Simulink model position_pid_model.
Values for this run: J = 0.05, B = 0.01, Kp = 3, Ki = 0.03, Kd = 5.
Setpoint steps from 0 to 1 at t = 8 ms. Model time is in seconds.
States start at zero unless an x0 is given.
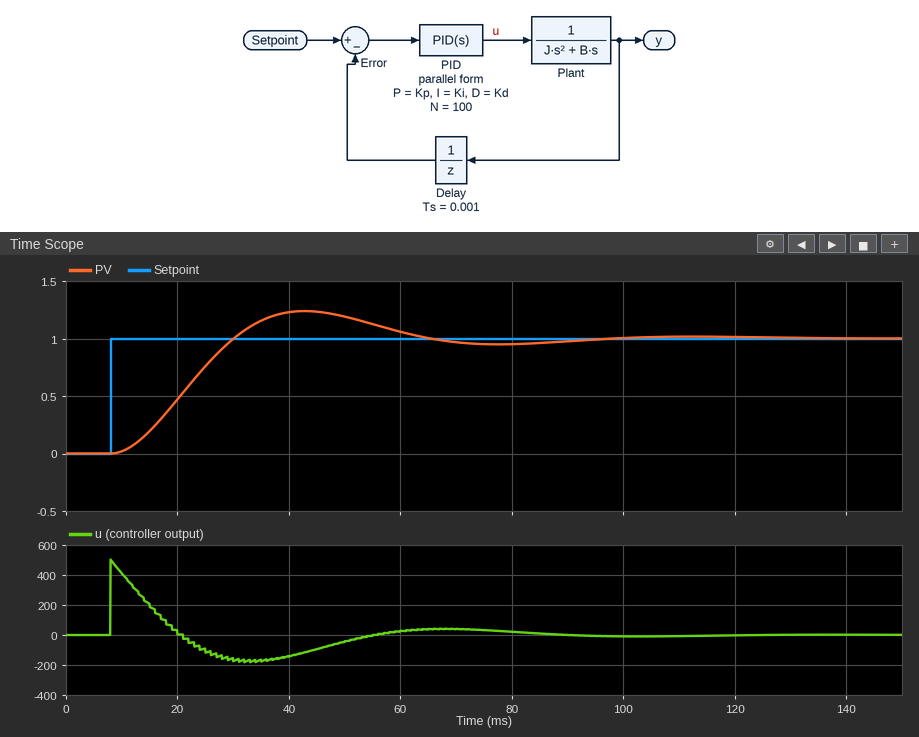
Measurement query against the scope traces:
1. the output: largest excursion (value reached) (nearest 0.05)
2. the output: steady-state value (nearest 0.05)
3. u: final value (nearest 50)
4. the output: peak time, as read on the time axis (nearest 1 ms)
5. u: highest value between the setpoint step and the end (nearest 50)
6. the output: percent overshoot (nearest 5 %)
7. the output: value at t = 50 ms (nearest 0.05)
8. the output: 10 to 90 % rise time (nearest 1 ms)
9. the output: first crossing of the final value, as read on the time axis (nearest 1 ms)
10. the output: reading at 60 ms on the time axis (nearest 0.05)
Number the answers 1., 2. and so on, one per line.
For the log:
1. 1.25
2. 1.00
3. 0
4. 43 ms
5. 500
6. 25 %
7. 1.20
8. 15 ms
9. 30 ms
10. 1.05
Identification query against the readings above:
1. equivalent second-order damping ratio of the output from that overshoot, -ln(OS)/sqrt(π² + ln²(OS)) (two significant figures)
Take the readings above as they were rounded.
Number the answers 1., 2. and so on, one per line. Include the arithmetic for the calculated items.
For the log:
1. ln(0.25) = -1.386; 1.386 / sqrt(9.870 + 1.922) = 0.40
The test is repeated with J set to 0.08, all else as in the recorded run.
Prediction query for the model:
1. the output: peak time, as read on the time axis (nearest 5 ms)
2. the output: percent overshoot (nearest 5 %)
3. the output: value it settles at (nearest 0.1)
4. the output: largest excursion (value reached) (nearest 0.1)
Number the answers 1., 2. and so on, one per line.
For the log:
1. 55 ms
2. 10 %
3. 1.0
4. 1.1
